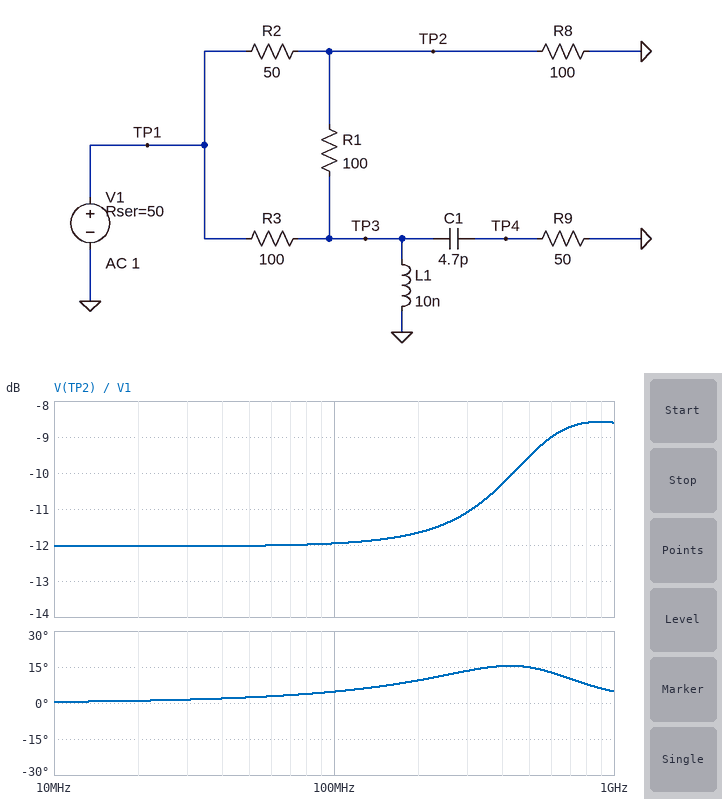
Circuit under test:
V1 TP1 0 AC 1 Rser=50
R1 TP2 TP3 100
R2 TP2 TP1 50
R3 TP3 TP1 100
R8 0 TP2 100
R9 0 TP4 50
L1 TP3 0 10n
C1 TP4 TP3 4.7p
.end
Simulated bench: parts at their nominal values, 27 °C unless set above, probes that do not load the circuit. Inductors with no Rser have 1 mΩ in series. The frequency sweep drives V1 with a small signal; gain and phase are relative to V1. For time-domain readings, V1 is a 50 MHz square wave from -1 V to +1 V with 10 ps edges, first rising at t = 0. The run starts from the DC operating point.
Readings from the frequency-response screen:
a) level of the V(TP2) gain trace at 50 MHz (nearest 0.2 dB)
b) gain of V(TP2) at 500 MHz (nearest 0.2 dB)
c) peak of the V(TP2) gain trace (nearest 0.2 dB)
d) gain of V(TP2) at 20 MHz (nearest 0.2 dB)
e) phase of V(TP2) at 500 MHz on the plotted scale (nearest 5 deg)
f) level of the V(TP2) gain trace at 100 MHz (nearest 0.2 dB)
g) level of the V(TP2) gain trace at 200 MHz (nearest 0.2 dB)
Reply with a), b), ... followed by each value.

a) -12.0 dB
b) -9.6 dB
c) -8.6 dB
d) -12.0 dB
e) 15 deg
f) -12.0 dB
g) -11.6 dB
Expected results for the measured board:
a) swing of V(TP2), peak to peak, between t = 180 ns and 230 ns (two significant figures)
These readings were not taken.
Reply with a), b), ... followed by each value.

a) 910 mV
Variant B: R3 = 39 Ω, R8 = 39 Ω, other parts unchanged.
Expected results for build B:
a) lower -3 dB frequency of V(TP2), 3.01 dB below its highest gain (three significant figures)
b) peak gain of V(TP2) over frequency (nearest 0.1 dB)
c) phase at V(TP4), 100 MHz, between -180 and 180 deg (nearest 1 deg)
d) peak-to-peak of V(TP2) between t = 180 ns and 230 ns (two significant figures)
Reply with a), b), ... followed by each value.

a) 287 MHz
b) -12.7 dB
c) 164 deg
d) 610 mV
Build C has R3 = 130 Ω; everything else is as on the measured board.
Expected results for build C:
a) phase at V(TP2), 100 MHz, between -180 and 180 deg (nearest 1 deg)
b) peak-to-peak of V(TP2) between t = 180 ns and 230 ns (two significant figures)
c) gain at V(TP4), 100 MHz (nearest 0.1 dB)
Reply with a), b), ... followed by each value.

a) 4 deg
b) 890 mV
c) -44.0 dB
